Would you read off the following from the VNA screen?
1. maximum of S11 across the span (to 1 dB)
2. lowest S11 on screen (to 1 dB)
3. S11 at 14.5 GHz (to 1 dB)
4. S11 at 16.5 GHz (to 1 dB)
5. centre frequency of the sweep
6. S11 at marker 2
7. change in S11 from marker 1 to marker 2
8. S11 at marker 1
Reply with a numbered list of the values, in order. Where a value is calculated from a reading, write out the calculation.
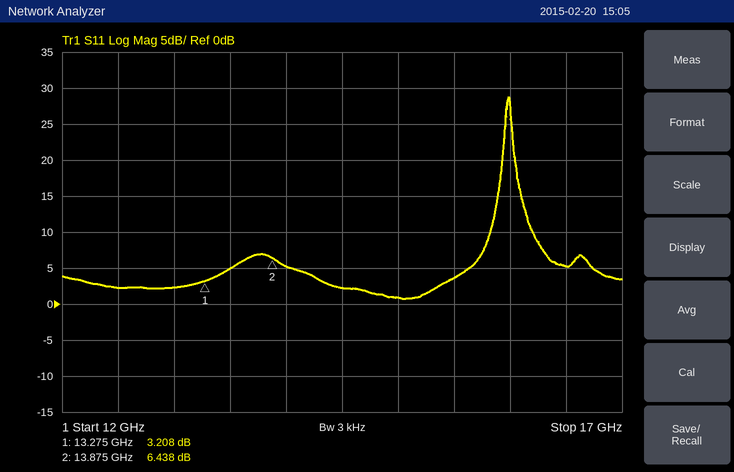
1. 29 dB
2. 1 dB
3. 2 dB
4. 5 dB
5. 14.5 GHz
6. 6.438 dB
7. 6.438 − (3.208) = 3.230 dB
8. 3.208 dB
